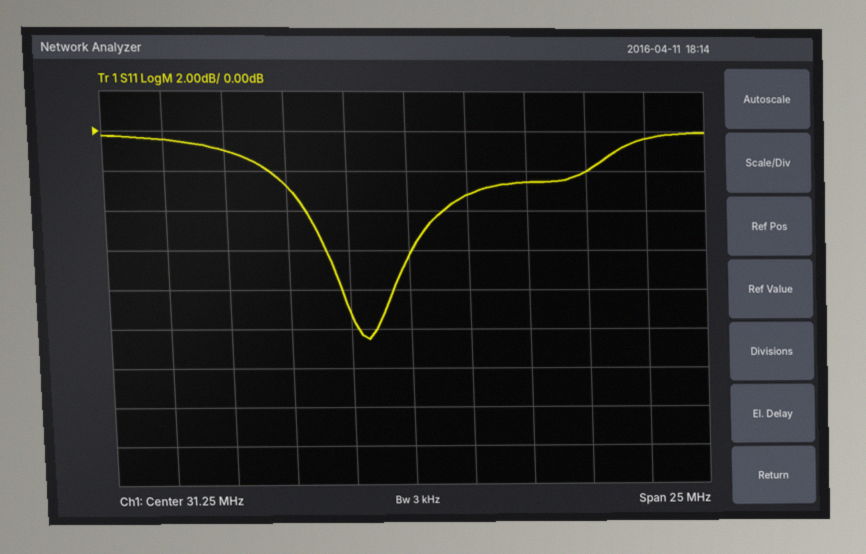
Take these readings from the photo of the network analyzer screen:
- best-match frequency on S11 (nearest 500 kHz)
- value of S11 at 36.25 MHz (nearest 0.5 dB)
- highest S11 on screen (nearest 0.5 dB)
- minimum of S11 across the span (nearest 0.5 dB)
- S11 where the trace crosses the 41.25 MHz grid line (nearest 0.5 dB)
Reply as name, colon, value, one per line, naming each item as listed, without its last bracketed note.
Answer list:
best-match frequency on S11: 29.5 MHz
value of S11 at 36.25 MHz: -2.5 dB
highest S11 on screen: 0.0 dB
minimum of S11 across the span: -10.5 dB
S11 where the trace crosses the 41.25 MHz grid line: -0.5 dB
